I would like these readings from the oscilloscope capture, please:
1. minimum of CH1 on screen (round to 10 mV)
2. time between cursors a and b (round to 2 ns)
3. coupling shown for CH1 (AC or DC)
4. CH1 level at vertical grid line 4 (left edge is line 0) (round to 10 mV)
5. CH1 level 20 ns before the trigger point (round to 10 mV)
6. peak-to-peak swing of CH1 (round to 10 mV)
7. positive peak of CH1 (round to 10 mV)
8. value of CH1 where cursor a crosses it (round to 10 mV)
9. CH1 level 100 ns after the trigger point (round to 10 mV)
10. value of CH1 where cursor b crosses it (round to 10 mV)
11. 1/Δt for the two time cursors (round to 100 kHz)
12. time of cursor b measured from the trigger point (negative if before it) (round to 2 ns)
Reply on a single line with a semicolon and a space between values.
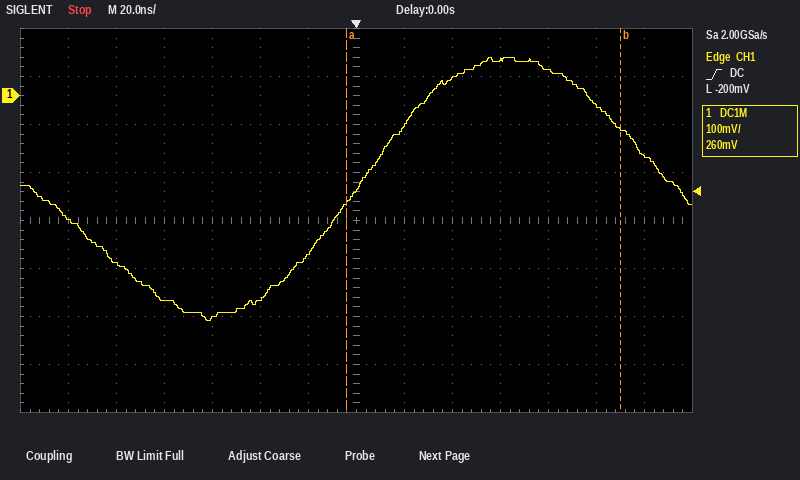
-470 mV; 114 ns; DC; -460 mV; -330 mV; 550 mV; 80 mV; -220 mV; -20 mV; -70 mV; 8.8 MHz; +110 ns
